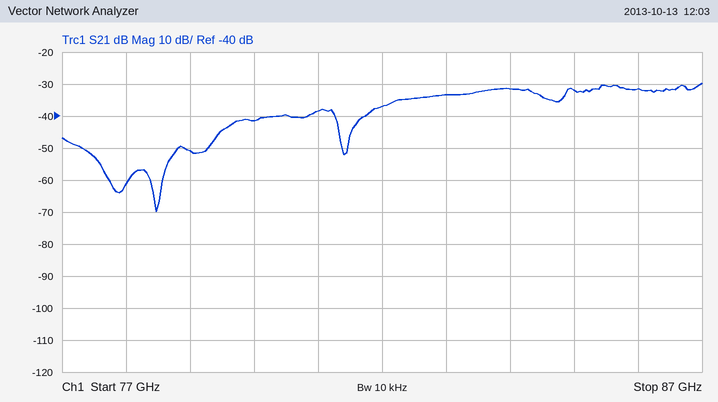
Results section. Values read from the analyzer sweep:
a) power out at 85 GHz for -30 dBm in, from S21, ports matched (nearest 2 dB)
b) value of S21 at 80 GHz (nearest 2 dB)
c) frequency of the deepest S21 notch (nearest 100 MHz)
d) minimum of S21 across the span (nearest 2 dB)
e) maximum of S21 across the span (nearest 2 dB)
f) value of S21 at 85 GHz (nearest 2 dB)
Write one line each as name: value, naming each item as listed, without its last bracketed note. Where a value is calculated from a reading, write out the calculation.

power out at 85 GHz for -30 dBm in, from S21, ports matched: -30 dBm + (-32 dB) = -62 dBm
value of S21 at 80 GHz: -42 dB
frequency of the deepest S21 notch: 78.5 GHz
minimum of S21 across the span: -70 dB
maximum of S21 across the span: -30 dB
value of S21 at 85 GHz: -32 dB
